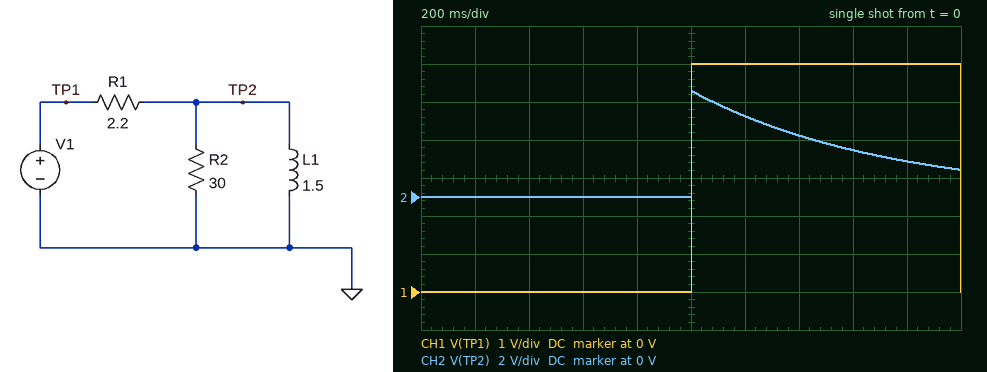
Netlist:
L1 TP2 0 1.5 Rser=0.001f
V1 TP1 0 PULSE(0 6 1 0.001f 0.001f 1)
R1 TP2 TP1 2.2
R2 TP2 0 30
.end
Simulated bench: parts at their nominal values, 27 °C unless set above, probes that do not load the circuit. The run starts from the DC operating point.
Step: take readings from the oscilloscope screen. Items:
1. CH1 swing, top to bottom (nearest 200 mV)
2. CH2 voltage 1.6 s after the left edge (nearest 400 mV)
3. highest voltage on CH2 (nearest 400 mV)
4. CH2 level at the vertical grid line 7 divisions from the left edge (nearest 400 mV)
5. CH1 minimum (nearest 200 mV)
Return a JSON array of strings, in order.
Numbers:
["6.0 V", "2.4 V", "5.6 V", "3.2 V", "0 V"]
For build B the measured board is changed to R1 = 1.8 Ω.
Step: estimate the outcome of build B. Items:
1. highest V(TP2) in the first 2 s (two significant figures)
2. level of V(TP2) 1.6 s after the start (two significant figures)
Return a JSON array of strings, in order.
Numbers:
["5.7 V", "2.9 V"]
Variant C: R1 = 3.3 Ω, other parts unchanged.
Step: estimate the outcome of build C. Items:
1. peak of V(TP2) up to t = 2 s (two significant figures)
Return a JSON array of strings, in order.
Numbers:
["5.4 V"]
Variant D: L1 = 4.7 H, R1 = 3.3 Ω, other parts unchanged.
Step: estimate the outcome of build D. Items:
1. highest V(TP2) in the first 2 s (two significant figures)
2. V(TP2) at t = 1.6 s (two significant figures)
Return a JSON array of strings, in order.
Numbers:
["5.4 V", "3.7 V"]
